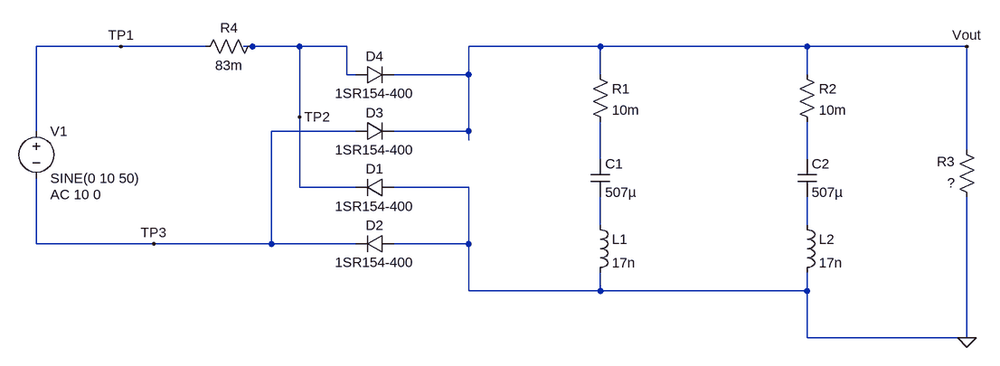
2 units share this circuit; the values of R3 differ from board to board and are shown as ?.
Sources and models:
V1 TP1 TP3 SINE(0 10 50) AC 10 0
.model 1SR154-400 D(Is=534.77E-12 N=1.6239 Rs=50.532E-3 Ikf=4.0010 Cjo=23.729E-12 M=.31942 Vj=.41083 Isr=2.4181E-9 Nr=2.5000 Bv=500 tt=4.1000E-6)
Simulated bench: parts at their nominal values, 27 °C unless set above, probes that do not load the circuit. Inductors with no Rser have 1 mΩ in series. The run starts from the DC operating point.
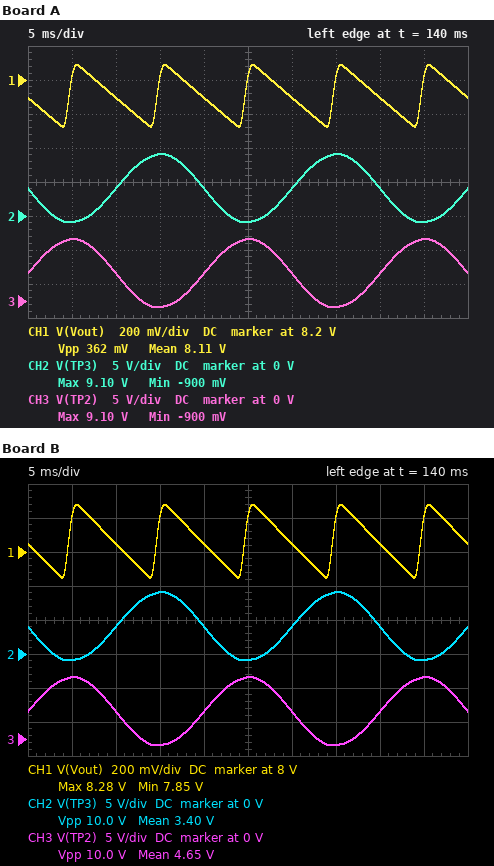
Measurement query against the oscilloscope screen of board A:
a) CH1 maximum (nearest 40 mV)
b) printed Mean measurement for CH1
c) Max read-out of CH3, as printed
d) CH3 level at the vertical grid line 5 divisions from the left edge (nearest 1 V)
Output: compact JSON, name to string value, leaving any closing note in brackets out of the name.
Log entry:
{"CH1 maximum": "8.28 V", "printed Mean measurement for CH1": "8.11 V", "Max read-out of CH3, as printed": "9.10 V", "CH3 level at the vertical grid line 5 divisions from the left edge": "9 V"}
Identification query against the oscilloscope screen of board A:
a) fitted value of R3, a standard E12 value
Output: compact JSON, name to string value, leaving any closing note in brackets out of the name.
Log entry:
{"fitted value of R3, a standard E12 value": "180 Ω"}
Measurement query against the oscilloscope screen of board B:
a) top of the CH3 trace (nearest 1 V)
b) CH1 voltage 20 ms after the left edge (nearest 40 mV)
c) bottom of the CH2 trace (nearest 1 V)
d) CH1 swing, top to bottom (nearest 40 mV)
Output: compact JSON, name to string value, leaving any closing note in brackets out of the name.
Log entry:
{"top of the CH3 trace": "9 V", "CH1 voltage 20 ms after the left edge": "8.04 V", "bottom of the CH2 trace": "-1 V", "CH1 swing, top to bottom": "440 mV"}
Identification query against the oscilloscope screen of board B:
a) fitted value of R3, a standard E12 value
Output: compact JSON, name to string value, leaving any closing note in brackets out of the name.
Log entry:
{"fitted value of R3, a standard E12 value": "150 Ω"}
